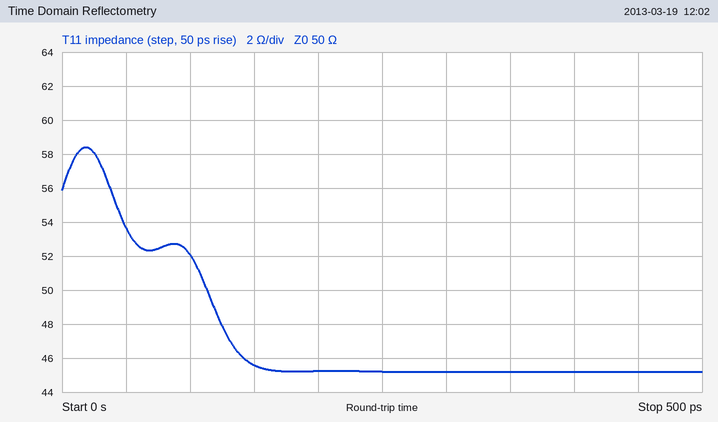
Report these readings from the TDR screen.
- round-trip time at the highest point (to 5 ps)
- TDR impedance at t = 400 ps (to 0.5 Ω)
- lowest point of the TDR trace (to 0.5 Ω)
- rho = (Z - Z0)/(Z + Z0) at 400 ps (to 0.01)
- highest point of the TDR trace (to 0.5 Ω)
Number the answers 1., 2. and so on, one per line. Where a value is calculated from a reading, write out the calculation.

1. 20 ps
2. 45.0 Ω
3. 45.0 Ω
4. (45 − 50)/(45 + 50) ≈ -0.05
5. 58.5 Ω
